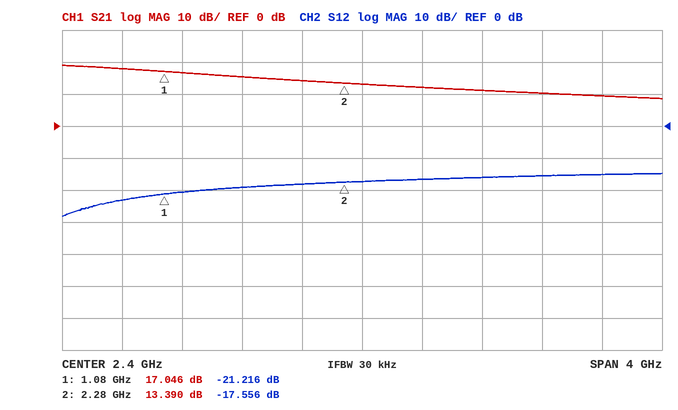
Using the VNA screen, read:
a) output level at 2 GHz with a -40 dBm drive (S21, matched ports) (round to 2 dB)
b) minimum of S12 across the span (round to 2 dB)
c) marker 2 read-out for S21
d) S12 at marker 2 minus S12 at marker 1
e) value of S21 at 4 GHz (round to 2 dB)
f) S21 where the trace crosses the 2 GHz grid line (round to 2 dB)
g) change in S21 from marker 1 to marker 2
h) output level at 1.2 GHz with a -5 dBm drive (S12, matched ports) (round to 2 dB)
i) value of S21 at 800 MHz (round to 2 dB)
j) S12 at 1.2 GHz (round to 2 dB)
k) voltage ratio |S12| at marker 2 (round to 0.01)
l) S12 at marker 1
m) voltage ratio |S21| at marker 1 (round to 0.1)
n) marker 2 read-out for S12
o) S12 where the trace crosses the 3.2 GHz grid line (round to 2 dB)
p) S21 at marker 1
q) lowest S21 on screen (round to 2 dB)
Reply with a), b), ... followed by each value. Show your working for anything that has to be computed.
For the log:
a) -40 dBm + (14 dB) = -26 dBm
b) -28 dB
c) 13.390 dB
d) -17.556 − (-21.216) = 3.660 dB
e) 10 dB
f) 14 dB
g) 13.39 − (17.046) = -3.656 dB
h) -5 dBm + (-20 dB) = -26 dBm
i) 18 dB
j) -20 dB
k) 10^(-17.556/20) ≈ 0.13
l) -21.216 dB
m) 10^(17.046/20) ≈ 7.1
n) -17.556 dB
o) -16 dB
p) 17.046 dB
q) 8 dB
